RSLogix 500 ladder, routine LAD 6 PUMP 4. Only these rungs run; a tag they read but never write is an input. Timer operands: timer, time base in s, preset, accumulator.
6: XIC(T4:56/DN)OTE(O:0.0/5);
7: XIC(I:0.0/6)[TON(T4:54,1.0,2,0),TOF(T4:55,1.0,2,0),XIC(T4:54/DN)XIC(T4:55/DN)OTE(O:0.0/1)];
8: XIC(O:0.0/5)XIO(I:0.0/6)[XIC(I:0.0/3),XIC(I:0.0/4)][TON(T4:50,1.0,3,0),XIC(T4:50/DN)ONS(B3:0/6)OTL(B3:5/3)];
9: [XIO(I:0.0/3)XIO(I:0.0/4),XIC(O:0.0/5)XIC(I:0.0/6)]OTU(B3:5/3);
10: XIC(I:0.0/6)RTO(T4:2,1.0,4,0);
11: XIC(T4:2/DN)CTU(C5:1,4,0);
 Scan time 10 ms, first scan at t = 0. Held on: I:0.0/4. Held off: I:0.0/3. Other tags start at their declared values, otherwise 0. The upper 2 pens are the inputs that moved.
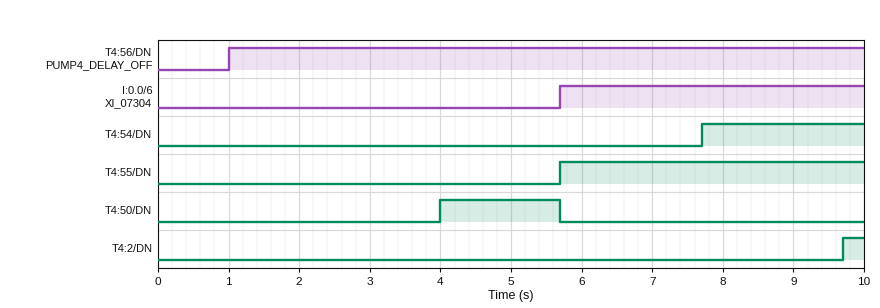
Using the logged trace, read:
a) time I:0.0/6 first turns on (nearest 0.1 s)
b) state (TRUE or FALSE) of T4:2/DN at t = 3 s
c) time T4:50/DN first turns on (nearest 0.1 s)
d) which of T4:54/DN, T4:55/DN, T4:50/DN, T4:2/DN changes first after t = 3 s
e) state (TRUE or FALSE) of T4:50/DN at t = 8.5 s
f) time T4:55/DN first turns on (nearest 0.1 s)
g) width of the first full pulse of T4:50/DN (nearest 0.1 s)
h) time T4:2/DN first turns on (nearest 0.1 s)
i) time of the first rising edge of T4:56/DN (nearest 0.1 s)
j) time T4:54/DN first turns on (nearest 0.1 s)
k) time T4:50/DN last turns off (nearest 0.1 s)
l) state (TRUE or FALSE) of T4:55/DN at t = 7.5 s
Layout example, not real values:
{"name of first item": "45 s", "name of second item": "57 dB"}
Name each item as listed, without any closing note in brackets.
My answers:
{"time I:0.0/6 first turns on": "5.7 s", "state (TRUE or FALSE) of T4:2/DN at t = 3 s": "FALSE", "time T4:50/DN first turns on": "4.0 s", "which of T4:54/DN, T4:55/DN, T4:50/DN, T4:2/DN changes first after t = 3 s": "T4:50/DN", "state (TRUE or FALSE) of T4:50/DN at t = 8.5 s": "FALSE", "time T4:55/DN first turns on": "5.7 s", "width of the first full pulse of T4:50/DN": "1.7 s", "time T4:2/DN first turns on": "9.7 s", "time of the first rising edge of T4:56/DN": "1.0 s", "time T4:54/DN first turns on": "7.7 s", "time T4:50/DN last turns off": "5.7 s", "state (TRUE or FALSE) of T4:55/DN at t = 7.5 s": "TRUE"}
